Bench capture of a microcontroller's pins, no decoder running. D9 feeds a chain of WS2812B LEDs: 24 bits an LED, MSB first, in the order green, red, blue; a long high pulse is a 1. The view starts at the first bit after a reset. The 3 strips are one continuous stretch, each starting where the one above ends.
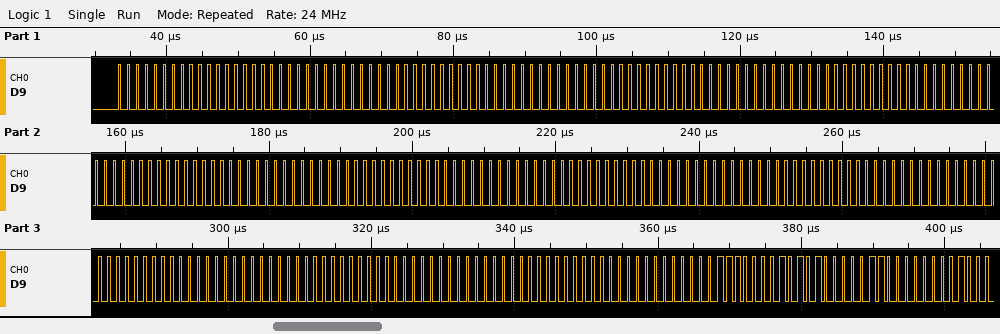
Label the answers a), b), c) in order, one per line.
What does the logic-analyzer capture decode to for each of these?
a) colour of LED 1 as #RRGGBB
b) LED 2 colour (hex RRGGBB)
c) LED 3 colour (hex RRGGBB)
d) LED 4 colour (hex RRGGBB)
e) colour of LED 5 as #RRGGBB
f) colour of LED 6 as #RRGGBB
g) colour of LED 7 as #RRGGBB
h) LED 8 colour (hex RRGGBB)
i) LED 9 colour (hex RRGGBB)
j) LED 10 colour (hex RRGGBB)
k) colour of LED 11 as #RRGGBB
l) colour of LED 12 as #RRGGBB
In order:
a) #000000
b) #000000
c) #000000
d) #000000
e) #000000
f) #000000
g) #000000
h) #000000
i) #000000
j) #000000
k) #000000
l) #150E06
